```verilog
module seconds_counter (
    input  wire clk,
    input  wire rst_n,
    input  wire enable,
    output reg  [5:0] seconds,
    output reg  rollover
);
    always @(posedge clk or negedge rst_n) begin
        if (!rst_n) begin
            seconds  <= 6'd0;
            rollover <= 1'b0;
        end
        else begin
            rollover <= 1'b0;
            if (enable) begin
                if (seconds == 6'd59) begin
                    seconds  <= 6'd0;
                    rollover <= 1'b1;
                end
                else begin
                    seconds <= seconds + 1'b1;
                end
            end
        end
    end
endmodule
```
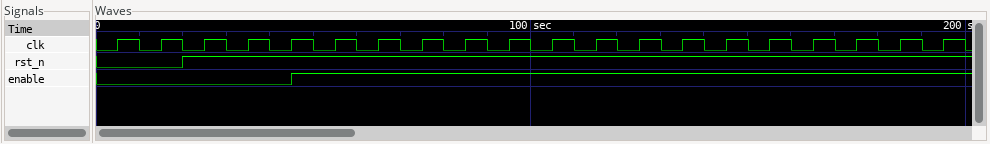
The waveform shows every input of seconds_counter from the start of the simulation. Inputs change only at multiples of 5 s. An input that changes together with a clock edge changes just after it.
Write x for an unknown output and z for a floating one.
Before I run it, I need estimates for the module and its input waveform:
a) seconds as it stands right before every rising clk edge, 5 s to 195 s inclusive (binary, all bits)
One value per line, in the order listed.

000000, 000000, 000000, 000000, 000000, 000000, 000001, 000010, 000011, 000100, 000101, 000110, 000111, 001000, 001001, 001010, 001011, 001100, 001101, 001110
